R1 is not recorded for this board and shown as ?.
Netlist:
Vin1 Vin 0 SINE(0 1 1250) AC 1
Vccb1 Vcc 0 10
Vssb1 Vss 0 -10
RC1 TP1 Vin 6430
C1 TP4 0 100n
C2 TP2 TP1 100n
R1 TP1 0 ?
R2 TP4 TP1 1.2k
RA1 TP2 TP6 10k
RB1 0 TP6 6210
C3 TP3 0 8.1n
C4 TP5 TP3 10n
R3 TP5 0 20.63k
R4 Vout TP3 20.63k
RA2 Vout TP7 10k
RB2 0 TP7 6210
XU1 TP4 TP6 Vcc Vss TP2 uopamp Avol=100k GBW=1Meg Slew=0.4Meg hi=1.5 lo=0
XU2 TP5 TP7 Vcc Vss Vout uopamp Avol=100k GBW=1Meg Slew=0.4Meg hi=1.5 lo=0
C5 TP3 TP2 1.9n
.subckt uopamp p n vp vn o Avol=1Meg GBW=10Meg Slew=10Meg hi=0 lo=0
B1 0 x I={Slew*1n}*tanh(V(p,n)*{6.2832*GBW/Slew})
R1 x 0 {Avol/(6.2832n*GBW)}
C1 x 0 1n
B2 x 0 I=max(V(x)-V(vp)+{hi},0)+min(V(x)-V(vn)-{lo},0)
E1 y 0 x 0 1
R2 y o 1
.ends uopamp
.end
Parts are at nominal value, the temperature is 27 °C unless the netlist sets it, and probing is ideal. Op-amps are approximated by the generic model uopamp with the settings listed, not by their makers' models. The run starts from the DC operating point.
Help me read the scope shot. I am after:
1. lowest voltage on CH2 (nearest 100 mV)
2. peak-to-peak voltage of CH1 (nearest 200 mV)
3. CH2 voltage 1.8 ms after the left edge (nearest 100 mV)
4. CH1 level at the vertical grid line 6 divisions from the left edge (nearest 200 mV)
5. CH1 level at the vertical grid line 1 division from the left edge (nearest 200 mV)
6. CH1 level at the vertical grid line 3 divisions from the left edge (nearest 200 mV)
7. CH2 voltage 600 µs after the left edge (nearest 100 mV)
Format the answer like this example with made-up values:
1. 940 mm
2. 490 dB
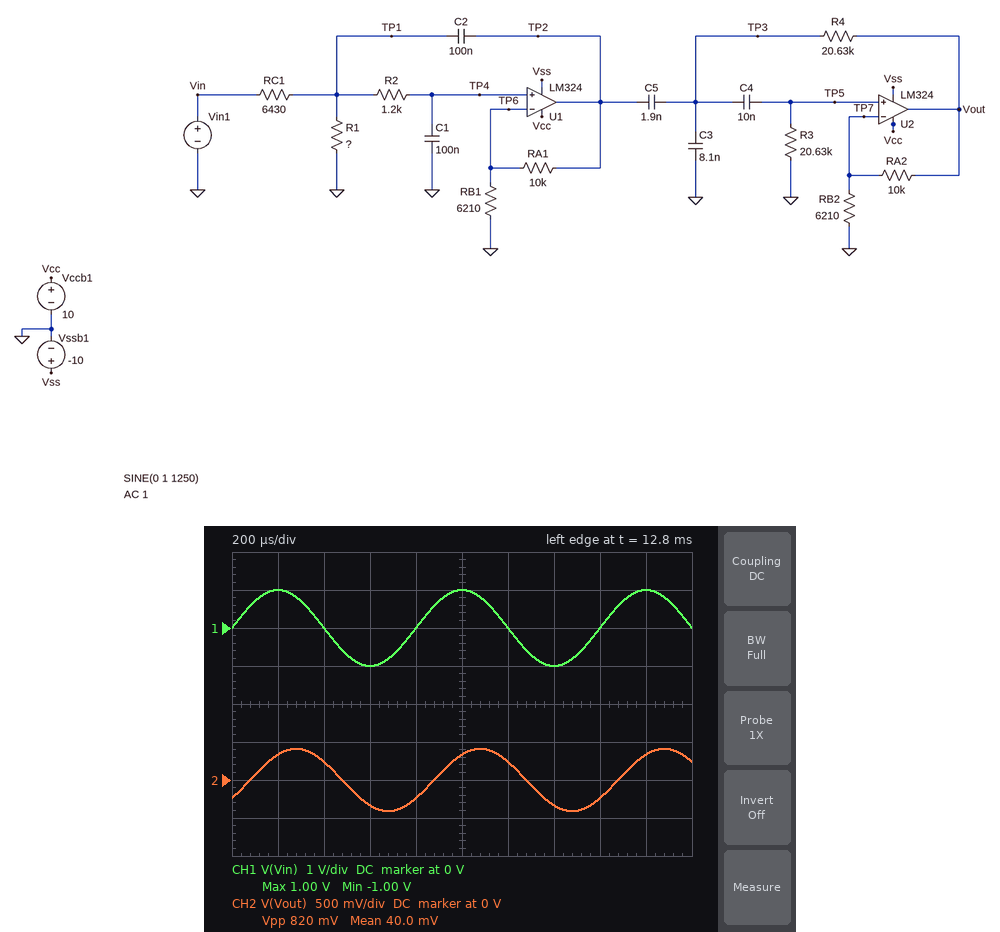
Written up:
1. -400 mV
2. 2.0 V
3. 300 mV
4. 0 V
5. 1.0 V
6. -1.0 V
7. -300 mV
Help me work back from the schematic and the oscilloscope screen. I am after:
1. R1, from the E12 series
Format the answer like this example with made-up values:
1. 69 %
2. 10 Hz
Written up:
1. 1 kΩ
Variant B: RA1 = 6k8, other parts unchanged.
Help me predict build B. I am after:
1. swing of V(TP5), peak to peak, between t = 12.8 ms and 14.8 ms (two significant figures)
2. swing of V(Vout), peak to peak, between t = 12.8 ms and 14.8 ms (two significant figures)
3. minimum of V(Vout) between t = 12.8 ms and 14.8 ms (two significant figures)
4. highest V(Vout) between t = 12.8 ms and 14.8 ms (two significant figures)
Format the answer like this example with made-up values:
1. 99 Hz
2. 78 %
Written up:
1. 170 mV
2. 440 mV
3. -220 mV
4. 220 mV
